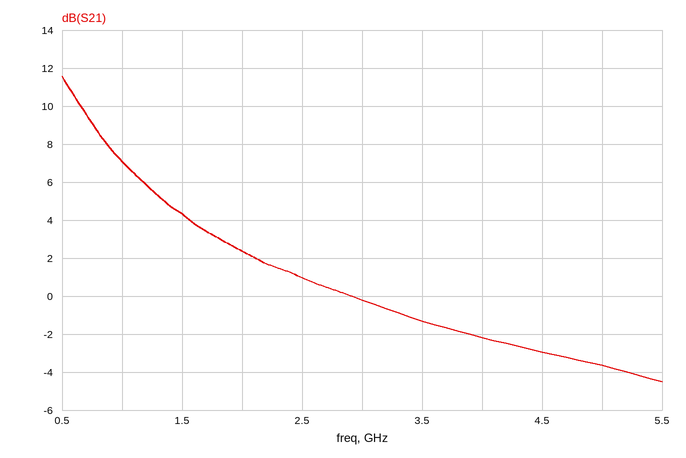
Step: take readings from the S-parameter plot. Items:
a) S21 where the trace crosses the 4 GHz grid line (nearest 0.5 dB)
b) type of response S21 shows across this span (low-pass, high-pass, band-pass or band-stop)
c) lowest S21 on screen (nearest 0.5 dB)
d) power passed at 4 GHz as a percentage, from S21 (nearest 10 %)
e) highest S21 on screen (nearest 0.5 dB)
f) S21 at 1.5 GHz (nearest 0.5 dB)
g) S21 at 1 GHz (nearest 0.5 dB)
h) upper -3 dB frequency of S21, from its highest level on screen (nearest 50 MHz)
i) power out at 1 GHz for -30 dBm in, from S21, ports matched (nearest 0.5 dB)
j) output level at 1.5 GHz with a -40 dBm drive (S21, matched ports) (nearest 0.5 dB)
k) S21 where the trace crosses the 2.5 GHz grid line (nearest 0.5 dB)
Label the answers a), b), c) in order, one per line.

a) -2.0 dB
b) low-pass
c) -4.5 dB
d) 60 %
e) 11.5 dB
f) 4.5 dB
g) 7.0 dB
h) 800 MHz
i) -23.0 dBm
j) -35.5 dBm
k) 1.0 dB
